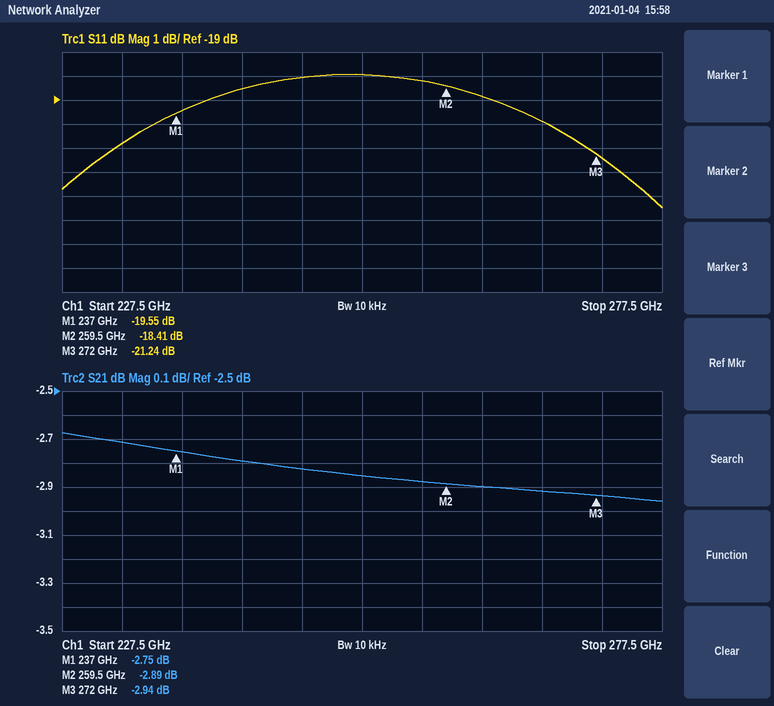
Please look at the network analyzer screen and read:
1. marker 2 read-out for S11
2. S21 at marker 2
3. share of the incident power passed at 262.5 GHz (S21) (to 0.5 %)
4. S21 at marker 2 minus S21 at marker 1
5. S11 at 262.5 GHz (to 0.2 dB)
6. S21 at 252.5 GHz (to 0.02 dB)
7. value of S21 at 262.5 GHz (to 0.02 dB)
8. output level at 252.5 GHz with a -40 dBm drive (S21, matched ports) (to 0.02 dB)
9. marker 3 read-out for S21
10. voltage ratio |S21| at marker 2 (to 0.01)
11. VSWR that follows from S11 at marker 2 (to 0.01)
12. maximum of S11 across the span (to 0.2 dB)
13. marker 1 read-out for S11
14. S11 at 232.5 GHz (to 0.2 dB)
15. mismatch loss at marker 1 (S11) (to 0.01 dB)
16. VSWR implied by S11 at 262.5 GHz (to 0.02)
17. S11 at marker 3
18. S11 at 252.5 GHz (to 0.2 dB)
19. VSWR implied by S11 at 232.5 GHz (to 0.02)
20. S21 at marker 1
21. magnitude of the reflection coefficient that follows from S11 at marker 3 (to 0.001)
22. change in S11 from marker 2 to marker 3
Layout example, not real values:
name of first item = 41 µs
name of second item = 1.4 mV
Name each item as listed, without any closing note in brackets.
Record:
marker 2 read-out for S11 = -18.41 dB
S21 at marker 2 = -2.89 dB
share of the incident power passed at 262.5 GHz (S21) = 51.5 %
S21 at marker 2 minus S21 at marker 1 = -0.14 dB
S11 at 262.5 GHz = -18.8 dB
S21 at 252.5 GHz = -2.86 dB
value of S21 at 262.5 GHz = -2.90 dB
output level at 252.5 GHz with a -40 dBm drive (S21, matched ports) = -42.86 dBm
marker 3 read-out for S21 = -2.94 dB
voltage ratio |S21| at marker 2 = 0.72
VSWR that follows from S11 at marker 2 = 1.27
maximum of S11 across the span = -18.0 dB
marker 1 read-out for S11 = -19.55 dB
S11 at 232.5 GHz = -20.8 dB
mismatch loss at marker 1 (S11) = 0.05 dB
VSWR implied by S11 at 262.5 GHz = 1.26
S11 at marker 3 = -21.24 dB
S11 at 252.5 GHz = -18.0 dB
VSWR implied by S11 at 232.5 GHz = 1.20
S21 at marker 1 = -2.75 dB
magnitude of the reflection coefficient that follows from S11 at marker 3 = 0.087
change in S11 from marker 2 to marker 3 = -2.83 dB
